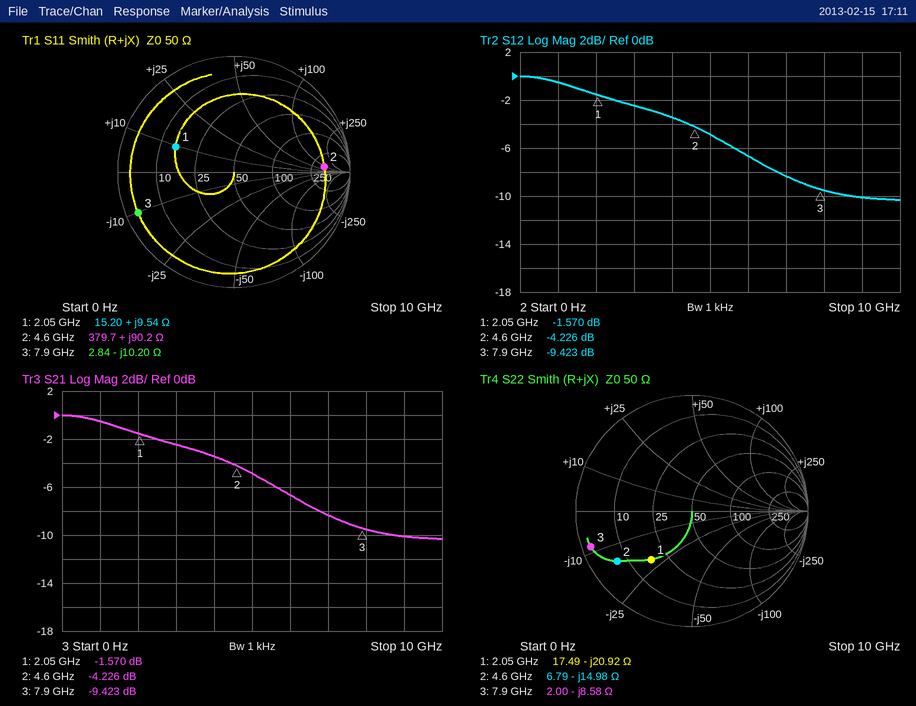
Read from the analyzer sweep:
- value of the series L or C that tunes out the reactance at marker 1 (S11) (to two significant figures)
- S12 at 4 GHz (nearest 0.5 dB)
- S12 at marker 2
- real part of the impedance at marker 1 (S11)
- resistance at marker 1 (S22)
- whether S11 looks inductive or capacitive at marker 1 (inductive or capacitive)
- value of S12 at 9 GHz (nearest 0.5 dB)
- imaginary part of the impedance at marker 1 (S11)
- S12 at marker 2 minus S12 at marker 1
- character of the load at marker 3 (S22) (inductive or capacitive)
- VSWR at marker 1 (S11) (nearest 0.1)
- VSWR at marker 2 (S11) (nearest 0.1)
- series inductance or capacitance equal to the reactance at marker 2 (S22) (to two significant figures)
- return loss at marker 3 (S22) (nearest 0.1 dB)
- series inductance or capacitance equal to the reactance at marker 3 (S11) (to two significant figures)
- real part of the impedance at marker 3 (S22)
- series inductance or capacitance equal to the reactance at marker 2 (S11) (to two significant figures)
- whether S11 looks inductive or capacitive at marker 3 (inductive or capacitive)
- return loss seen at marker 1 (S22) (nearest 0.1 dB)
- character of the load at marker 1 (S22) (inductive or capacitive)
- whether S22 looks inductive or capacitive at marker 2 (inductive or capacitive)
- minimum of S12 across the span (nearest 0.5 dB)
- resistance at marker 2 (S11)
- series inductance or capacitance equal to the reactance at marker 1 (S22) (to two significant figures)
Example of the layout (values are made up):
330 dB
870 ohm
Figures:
8.1 pF
-3.5 dB
-4.226 dB
15.20 Ω
17.49 Ω
inductive
-10.0 dB
+9.54 Ω
-2.656 dB
capacitive
3.4
8.0
2.3 pF
0.7 dB
2.0 pF
2.00 Ω
3.1 nH
capacitive
5.2 dB
capacitive
capacitive
-10.5 dB
379.7 Ω
3.7 pF
